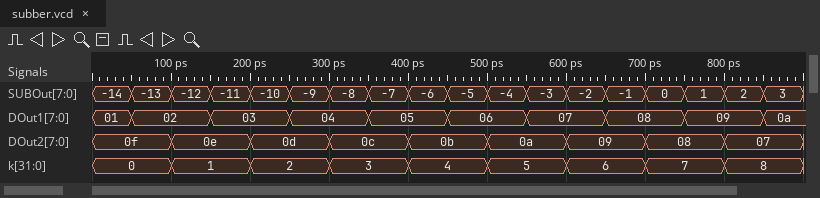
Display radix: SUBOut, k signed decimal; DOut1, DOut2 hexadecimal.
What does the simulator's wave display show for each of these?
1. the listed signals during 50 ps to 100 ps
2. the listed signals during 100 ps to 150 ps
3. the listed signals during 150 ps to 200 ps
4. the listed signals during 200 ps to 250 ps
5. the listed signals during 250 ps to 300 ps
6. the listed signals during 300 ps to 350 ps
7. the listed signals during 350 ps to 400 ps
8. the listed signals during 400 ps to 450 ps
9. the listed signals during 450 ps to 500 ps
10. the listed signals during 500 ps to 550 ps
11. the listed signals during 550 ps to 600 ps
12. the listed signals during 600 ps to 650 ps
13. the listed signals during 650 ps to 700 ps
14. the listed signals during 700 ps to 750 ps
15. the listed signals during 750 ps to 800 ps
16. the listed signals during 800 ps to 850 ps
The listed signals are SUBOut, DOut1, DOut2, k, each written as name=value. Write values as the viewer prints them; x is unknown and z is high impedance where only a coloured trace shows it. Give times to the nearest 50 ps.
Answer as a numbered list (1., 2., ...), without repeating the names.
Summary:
1. SUBOut=-13, DOut1=02, DOut2=0f, k=0
2. SUBOut=-12, DOut1=02, DOut2=0e, k=1
3. SUBOut=-11, DOut1=03, DOut2=0e, k=1
4. SUBOut=-10, DOut1=03, DOut2=0d, k=2
5. SUBOut=-9, DOut1=04, DOut2=0d, k=2
6. SUBOut=-8, DOut1=04, DOut2=0c, k=3
7. SUBOut=-7, DOut1=05, DOut2=0c, k=3
8. SUBOut=-6, DOut1=05, DOut2=0b, k=4
9. SUBOut=-5, DOut1=06, DOut2=0b, k=4
10. SUBOut=-4, DOut1=06, DOut2=0a, k=5
11. SUBOut=-3, DOut1=07, DOut2=0a, k=5
12. SUBOut=-2, DOut1=07, DOut2=09, k=6
13. SUBOut=-1, DOut1=08, DOut2=09, k=6
14. SUBOut=0, DOut1=08, DOut2=08, k=7
15. SUBOut=1, DOut1=09, DOut2=08, k=7
16. SUBOut=2, DOut1=09, DOut2=07, k=8
